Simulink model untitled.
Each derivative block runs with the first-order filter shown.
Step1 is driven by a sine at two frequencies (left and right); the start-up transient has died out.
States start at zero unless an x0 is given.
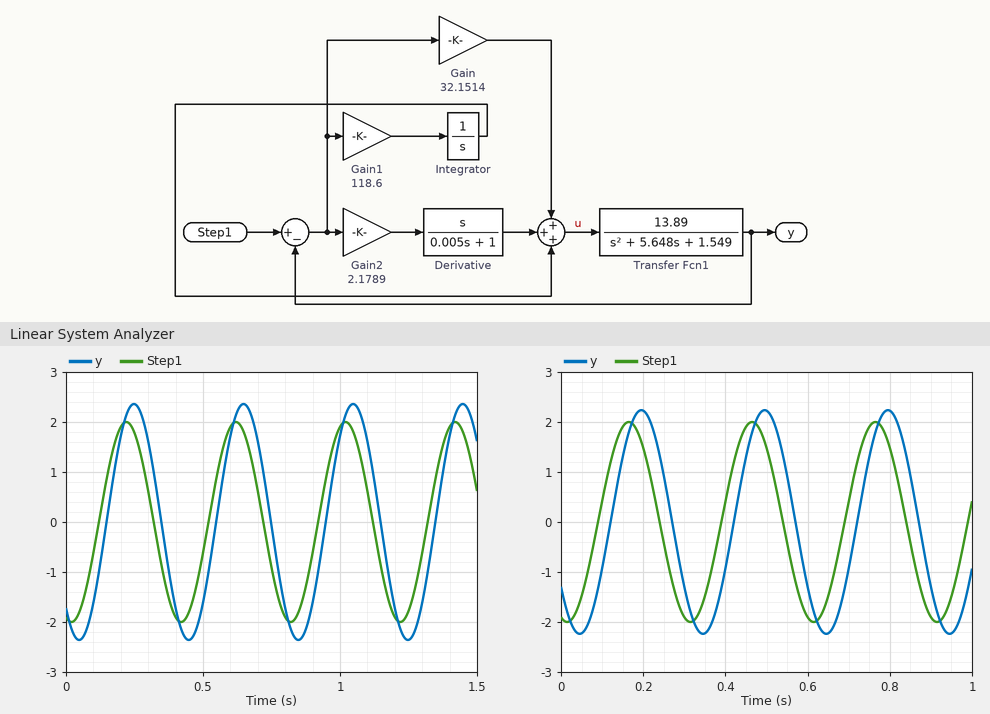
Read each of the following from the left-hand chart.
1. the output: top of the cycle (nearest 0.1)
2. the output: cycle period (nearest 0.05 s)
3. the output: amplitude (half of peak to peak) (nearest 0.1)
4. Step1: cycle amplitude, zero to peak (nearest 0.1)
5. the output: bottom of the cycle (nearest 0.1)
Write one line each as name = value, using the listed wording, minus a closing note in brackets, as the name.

the output: top of the cycle = 2.4
the output: cycle period = 0.40 s
the output: amplitude (half of peak to peak) = 2.4
Step1: cycle amplitude, zero to peak = 2.0
the output: bottom of the cycle = -2.4
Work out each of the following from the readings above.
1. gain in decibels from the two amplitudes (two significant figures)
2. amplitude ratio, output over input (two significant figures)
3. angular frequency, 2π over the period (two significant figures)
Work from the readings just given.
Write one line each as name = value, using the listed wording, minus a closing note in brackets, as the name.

gain in decibels from the two amplitudes = 1.6 dB
amplitude ratio, output over input = 1.2
angular frequency, 2π over the period = 16 rad/s
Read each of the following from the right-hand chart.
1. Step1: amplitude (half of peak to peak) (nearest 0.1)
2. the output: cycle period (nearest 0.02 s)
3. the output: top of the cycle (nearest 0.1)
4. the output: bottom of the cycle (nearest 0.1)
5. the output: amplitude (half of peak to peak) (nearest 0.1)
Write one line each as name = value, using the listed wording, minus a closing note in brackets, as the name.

Step1: amplitude (half of peak to peak) = 2.0
the output: cycle period = 0.30 s
the output: top of the cycle = 2.2
the output: bottom of the cycle = -2.2
the output: amplitude (half of peak to peak) = 2.2
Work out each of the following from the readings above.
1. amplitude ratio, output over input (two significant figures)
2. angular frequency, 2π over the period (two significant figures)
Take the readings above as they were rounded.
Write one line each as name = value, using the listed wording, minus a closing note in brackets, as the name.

amplitude ratio, output over input = 1.1
angular frequency, 2π over the period = 21 rad/s
